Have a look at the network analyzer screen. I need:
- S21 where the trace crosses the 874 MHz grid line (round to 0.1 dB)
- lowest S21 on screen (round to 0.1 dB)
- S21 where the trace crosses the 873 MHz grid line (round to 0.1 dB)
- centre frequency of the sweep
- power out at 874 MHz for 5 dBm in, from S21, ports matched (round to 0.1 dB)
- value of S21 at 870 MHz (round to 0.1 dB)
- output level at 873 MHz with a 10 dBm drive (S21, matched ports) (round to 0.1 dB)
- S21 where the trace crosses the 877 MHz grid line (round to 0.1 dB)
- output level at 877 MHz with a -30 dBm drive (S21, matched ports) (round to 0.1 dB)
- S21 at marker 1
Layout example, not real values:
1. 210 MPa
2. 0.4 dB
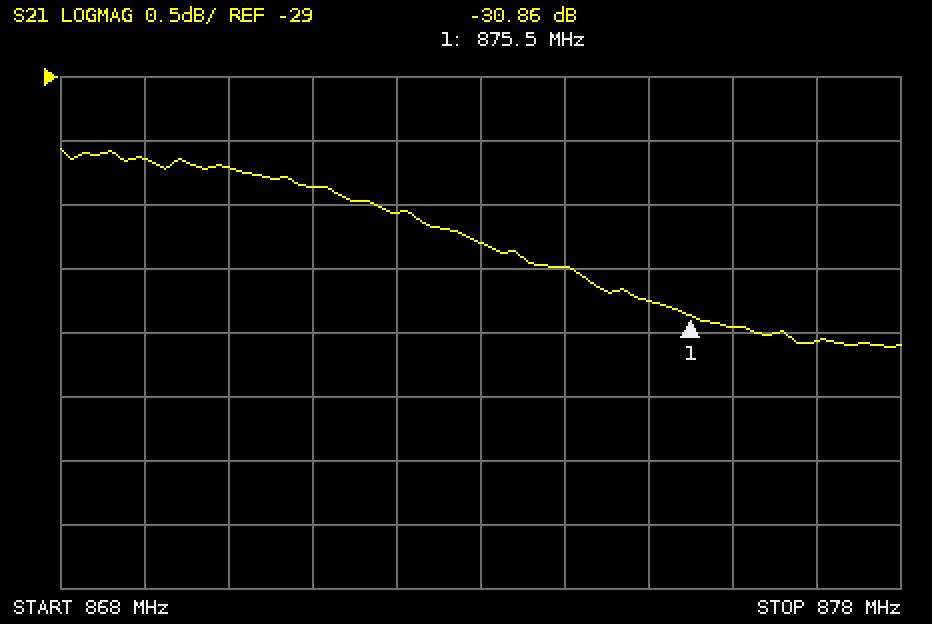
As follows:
1. -30.5 dB
2. -31.1 dB
3. -30.3 dB
4. 873 MHz
5. -25.5 dBm
6. -29.7 dB
7. -20.3 dBm
8. -31.1 dB
9. -61.1 dBm
10. -30.86 dB
